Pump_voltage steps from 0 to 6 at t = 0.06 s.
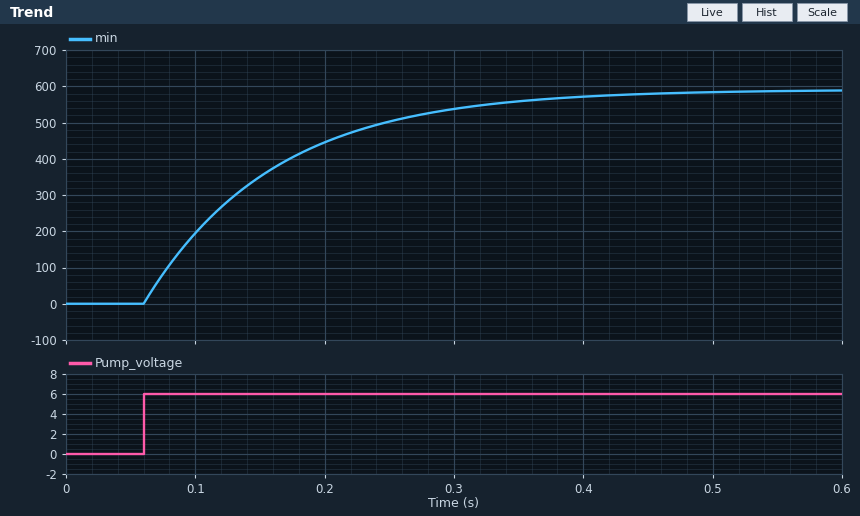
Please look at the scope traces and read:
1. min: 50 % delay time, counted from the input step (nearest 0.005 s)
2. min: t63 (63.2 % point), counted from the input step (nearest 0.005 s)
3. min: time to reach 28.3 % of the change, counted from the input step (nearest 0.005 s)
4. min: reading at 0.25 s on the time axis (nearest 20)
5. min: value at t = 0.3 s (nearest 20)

0.070 s
0.100 s
0.035 s
500
540
